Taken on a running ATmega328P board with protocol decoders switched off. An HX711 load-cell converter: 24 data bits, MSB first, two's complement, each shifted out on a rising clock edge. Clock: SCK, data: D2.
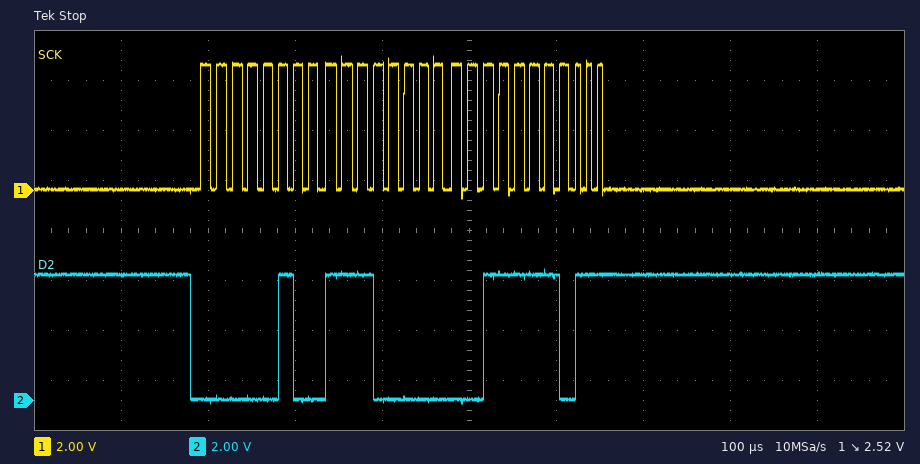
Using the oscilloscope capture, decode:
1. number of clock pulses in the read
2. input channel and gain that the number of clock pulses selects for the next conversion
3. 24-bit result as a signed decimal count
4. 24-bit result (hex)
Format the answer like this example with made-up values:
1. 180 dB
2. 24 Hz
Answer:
1. 27
2. channel A, gain 64
3. 319550
4. 0x04E03E
